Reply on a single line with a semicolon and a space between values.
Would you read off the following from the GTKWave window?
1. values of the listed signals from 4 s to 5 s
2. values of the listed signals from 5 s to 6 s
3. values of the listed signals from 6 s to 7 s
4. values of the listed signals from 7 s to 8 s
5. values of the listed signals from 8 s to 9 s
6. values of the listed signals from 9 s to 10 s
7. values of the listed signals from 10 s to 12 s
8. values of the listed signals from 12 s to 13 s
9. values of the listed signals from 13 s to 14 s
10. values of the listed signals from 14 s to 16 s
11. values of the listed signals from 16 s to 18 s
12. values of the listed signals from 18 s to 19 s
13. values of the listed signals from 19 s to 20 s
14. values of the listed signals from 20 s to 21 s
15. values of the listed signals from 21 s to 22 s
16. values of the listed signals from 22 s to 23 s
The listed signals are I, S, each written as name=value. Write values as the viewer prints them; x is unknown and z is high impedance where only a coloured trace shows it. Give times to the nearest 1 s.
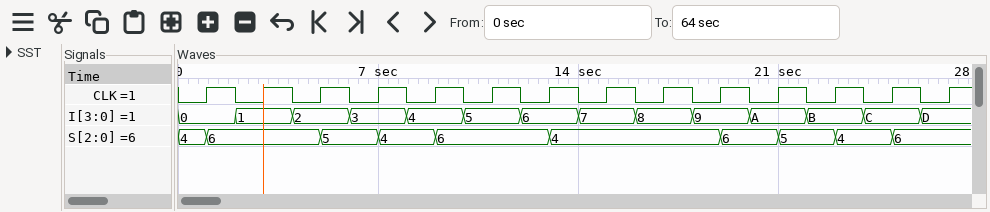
I=2, S=6; I=2, S=5; I=3, S=5; I=3, S=4; I=4, S=4; I=4, S=6; I=5, S=6; I=6, S=6; I=6, S=4; I=7, S=4; I=8, S=4; I=9, S=4; I=9, S=6; I=A, S=6; I=A, S=5; I=B, S=5
